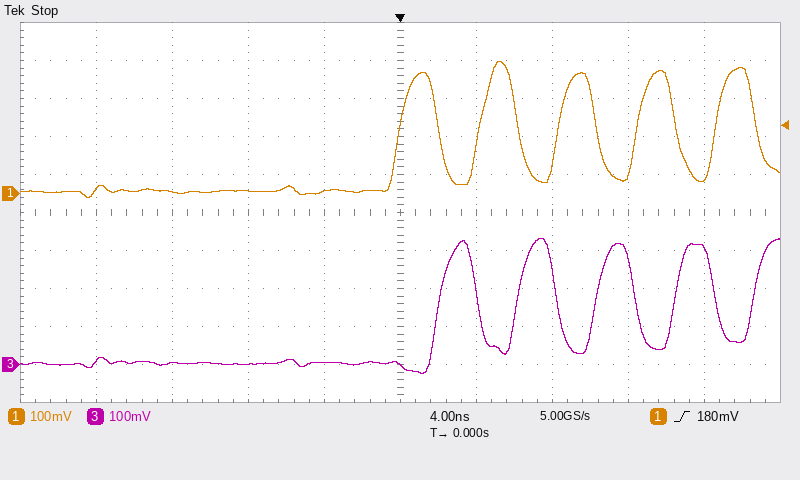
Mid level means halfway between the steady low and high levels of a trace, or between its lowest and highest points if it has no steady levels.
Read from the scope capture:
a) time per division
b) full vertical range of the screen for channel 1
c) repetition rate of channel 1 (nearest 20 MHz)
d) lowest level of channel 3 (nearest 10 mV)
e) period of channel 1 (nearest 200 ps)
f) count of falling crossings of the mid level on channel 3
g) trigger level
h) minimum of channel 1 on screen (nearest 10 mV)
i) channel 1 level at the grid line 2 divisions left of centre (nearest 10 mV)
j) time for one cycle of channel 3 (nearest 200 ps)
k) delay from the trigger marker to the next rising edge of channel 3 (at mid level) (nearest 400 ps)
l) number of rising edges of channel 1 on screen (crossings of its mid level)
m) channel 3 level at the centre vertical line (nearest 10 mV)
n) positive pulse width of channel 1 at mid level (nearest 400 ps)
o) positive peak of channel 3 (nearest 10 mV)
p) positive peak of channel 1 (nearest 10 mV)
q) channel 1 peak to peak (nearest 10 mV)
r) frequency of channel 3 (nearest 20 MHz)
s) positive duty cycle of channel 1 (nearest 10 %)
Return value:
4 ns
1 V
240 MHz
-20 mV
4.2 ns
4
180 mV
-10 mV
10 mV
4.2 ns
2.0 ns
5
0 mV
2.0 ns
330 mV
350 mV
360 mV
240 MHz
50 %
